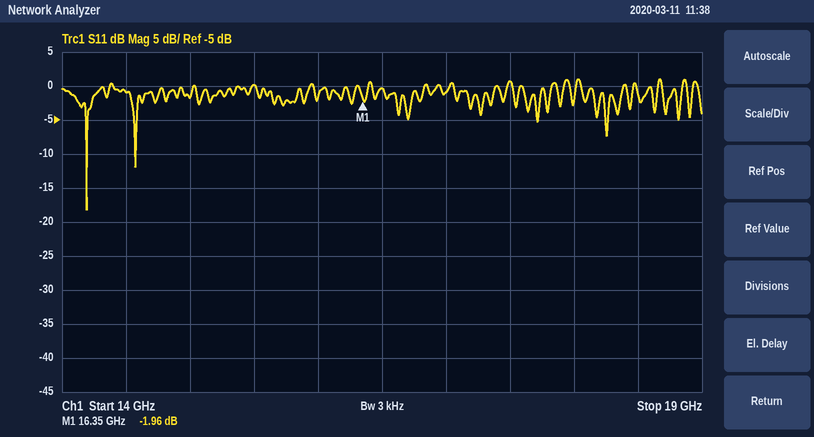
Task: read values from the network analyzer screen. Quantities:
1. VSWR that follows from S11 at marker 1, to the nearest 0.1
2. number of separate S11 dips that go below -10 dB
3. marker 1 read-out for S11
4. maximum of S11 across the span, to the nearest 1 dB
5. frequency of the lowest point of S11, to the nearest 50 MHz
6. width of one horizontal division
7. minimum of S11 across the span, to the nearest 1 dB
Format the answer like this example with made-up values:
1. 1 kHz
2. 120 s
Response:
1. 8.9
2. 2
3. -1.96 dB
4. 1 dB
5. 14.20 GHz
6. 500 MHz
7. -18 dB
